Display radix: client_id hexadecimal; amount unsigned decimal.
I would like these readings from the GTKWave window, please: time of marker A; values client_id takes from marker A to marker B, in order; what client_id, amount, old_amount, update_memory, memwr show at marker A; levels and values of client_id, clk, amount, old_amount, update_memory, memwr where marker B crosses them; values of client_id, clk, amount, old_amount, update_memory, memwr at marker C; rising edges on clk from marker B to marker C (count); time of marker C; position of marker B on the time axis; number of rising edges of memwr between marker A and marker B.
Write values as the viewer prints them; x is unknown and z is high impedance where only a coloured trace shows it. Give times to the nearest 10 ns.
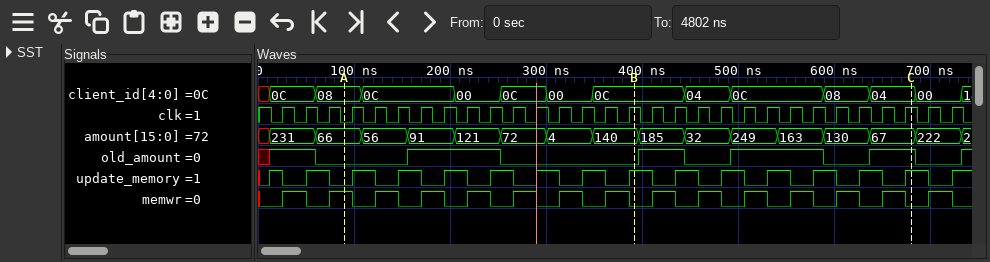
90 ns
08, 0C, 00, 0C, 00, 0C
client_id=08, amount=66, old_amount=0, update_memory=0, memwr=1
client_id=0C, clk=1, amount=140, old_amount=0, update_memory=1, memwr=0
client_id=04, clk=1, amount=67, old_amount=1, update_memory=1, memwr=0
12
680 ns
390 ns
6
